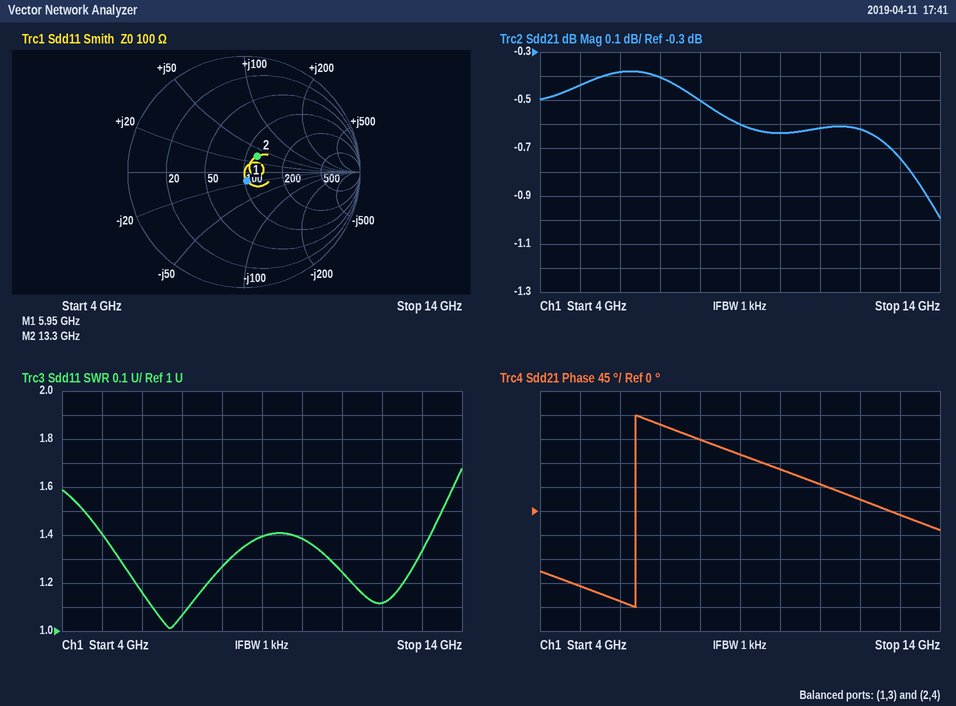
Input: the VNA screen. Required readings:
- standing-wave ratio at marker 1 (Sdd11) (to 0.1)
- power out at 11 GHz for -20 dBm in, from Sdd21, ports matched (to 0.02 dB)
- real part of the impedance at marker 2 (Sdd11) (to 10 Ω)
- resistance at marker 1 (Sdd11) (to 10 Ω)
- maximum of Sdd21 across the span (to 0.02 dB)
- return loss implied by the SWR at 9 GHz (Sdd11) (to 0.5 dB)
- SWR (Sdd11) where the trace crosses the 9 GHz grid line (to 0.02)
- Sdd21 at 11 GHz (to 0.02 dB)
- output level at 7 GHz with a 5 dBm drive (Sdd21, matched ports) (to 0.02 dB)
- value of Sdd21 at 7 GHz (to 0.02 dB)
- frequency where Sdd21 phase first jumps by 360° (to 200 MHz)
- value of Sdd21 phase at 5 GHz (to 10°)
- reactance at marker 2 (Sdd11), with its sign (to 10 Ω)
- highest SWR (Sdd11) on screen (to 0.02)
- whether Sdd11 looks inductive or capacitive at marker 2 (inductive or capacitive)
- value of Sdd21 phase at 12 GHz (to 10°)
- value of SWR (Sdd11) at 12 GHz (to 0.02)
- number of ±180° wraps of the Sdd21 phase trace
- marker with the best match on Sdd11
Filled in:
1.2
-20.62 dBm
120 Ω
100 Ω
-0.38 dB
15.5 dB
1.40
-0.62 dB
4.60 dBm
-0.40 dB
6.4 GHz
-140°
+30 Ω
1.68
inductive
20°
1.12
1
marker 1
